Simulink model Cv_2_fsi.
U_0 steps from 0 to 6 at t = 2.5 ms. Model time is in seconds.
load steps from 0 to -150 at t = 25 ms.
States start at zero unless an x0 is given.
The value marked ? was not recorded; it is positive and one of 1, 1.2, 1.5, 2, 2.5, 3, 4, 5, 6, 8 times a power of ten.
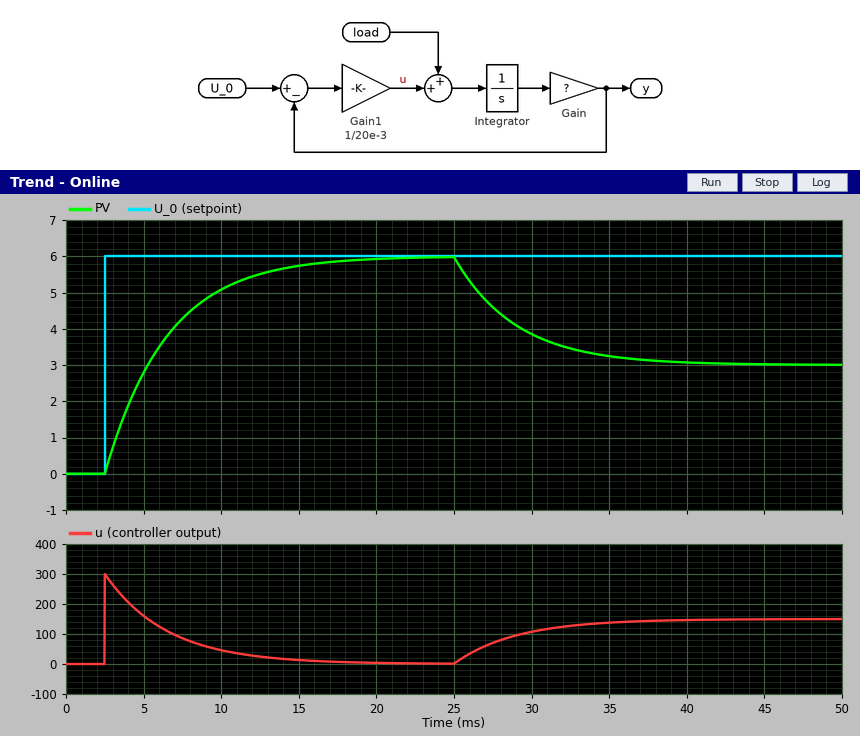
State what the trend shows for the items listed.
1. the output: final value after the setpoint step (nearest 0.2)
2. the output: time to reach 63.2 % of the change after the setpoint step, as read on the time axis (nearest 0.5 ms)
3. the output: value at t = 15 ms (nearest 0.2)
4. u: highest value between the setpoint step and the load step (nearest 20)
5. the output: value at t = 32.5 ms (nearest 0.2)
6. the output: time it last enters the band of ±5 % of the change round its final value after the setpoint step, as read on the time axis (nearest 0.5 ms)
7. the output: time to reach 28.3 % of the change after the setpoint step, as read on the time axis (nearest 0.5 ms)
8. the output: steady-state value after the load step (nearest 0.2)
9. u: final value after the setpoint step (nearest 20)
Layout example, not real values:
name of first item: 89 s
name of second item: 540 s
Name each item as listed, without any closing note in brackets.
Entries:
the output: final value after the setpoint step: 6.0
the output: time to reach 63.2 % of the change after the setpoint step, as read on the time axis: 6.5 ms
the output: value at t = 15 ms: 5.8
u: highest value between the setpoint step and the load step: 300
the output: value at t = 32.5 ms: 3.4
the output: time it last enters the band of ±5 % of the change round its final value after the setpoint step, as read on the time axis: 14.5 ms
the output: time to reach 28.3 % of the change after the setpoint step, as read on the time axis: 4.0 ms
the output: steady-state value after the load step: 3.0
u: final value after the setpoint step: 0
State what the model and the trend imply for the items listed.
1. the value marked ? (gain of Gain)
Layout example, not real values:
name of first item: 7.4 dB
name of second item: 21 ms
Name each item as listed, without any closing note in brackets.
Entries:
the value marked ?: 5
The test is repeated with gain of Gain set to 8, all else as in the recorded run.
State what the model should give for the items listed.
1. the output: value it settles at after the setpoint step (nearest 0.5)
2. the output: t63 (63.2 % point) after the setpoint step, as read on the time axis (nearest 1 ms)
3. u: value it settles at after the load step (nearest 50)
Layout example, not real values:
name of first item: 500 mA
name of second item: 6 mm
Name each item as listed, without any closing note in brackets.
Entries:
the output: value it settles at after the setpoint step: 6.0
the output: t63 (63.2 % point) after the setpoint step, as read on the time axis: 5 ms
u: value it settles at after the load step: 150
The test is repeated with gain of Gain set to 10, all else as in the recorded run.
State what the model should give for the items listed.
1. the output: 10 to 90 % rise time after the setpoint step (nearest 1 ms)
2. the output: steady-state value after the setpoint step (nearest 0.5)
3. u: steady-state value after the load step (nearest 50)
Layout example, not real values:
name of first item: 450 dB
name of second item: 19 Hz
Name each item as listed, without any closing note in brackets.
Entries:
the output: 10 to 90 % rise time after the setpoint step: 4 ms
the output: steady-state value after the setpoint step: 6.0
u: steady-state value after the load step: 150
